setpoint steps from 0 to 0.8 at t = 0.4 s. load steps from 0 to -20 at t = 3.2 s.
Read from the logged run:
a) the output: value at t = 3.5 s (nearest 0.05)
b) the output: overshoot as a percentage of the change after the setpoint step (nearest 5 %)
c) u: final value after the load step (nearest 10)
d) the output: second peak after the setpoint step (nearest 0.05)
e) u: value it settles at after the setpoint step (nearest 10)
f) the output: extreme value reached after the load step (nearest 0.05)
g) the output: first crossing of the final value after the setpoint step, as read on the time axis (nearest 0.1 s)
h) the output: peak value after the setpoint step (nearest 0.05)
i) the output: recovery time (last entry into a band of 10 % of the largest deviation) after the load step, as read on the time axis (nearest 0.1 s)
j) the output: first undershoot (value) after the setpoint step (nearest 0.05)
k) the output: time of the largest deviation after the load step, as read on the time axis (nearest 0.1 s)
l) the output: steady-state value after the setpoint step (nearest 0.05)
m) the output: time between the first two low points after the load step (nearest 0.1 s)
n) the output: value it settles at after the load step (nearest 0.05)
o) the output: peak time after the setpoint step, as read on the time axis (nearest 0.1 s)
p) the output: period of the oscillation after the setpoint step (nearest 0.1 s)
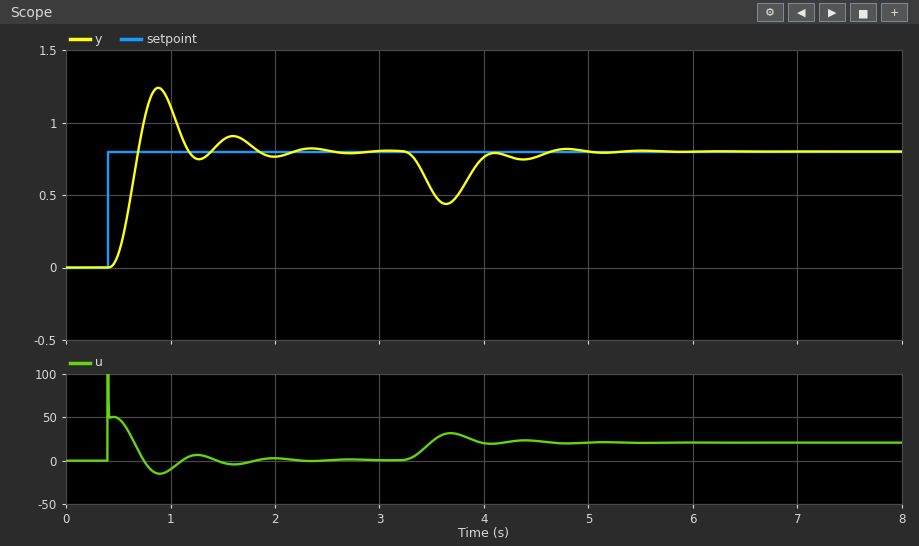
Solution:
0.55
55 %
20
0.90
0
0.45
0.7 s
1.25
4.5 s
0.75
3.6 s
0.80
0.7 s
0.80
0.9 s
0.7 s
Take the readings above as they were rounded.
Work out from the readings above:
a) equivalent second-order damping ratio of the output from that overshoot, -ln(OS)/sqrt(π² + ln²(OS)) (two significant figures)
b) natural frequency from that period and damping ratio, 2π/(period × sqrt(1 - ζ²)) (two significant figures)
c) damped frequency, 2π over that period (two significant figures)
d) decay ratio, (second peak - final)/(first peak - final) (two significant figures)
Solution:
0.19
9.1 rad/s
9.0 rad/s
0.22
